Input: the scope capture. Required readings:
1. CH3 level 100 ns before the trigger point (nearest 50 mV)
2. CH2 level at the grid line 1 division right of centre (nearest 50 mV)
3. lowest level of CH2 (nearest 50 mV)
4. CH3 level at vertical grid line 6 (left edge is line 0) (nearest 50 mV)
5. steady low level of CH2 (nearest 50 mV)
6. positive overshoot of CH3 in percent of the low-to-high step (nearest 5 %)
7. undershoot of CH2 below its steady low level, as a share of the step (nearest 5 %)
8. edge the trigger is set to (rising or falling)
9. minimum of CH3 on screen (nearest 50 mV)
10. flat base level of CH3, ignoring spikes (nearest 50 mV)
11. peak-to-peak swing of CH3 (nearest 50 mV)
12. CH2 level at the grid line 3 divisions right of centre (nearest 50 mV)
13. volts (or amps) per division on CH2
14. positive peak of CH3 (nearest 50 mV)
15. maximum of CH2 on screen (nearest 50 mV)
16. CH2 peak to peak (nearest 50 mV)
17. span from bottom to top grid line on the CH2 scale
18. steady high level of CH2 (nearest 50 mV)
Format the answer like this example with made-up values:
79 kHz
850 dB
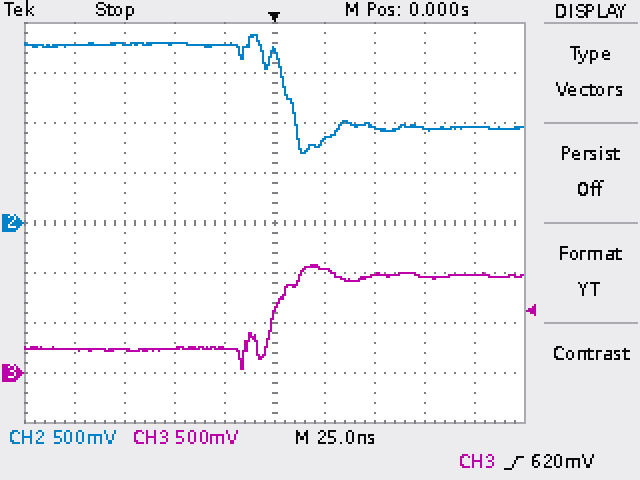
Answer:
250 mV
800 mV
700 mV
1.05 V
950 mV
15 %
30 %
rising
50 mV
250 mV
1.05 V
950 mV
500 mV
1.10 V
1.90 V
1.20 V
4 V
1.80 V
